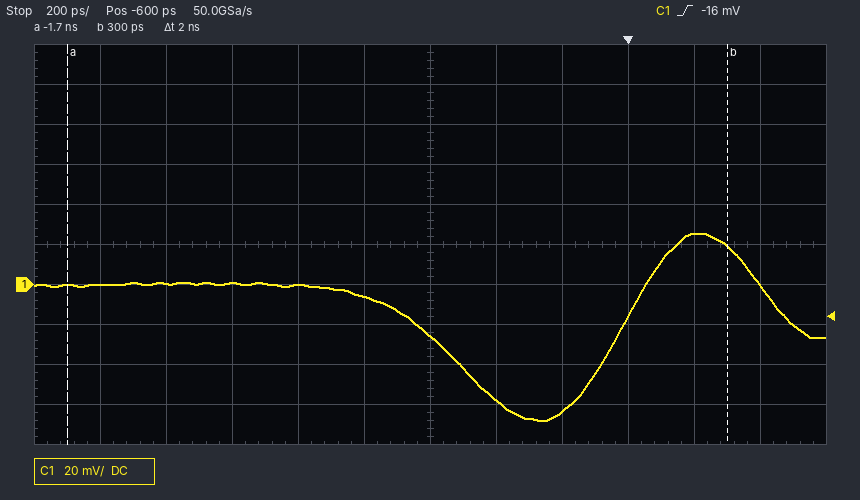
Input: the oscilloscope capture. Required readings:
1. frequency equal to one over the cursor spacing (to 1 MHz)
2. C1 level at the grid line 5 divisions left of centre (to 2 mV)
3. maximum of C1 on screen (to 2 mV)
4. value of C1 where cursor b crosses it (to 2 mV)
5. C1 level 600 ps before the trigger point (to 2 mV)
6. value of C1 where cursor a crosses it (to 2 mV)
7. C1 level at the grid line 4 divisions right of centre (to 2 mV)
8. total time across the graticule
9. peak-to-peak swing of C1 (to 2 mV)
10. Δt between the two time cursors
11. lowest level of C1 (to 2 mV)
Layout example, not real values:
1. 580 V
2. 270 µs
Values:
1. 500 MHz
2. 0 mV
3. 26 mV
4. 20 mV
5. -26 mV
6. 0 mV
7. 26 mV
8. 2.4 ns
9. 94 mV
10. 2 ns
11. -68 mV
